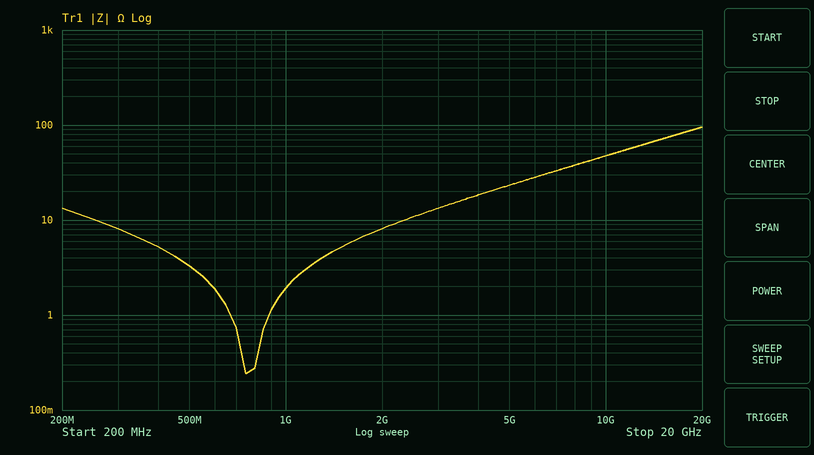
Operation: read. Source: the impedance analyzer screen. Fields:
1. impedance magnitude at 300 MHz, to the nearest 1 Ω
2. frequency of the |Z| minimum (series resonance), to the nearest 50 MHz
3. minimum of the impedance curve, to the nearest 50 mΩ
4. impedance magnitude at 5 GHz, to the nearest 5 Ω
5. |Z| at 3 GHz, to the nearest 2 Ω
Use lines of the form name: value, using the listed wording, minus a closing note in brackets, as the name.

impedance magnitude at 300 MHz, to the nearest 1 Ω: 8 Ω
frequency of the |Z| minimum (series resonance), to the nearest 50 MHz: 750 MHz
minimum of the impedance curve, to the nearest 50 mΩ: 250 mΩ
impedance magnitude at 5 GHz, to the nearest 5 Ω: 25 Ω
|Z| at 3 GHz, to the nearest 2 Ω: 14 Ω
